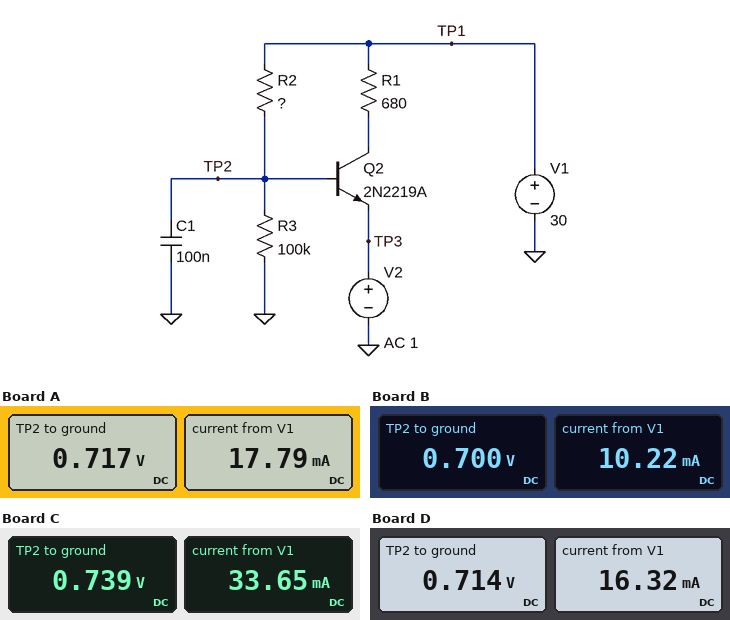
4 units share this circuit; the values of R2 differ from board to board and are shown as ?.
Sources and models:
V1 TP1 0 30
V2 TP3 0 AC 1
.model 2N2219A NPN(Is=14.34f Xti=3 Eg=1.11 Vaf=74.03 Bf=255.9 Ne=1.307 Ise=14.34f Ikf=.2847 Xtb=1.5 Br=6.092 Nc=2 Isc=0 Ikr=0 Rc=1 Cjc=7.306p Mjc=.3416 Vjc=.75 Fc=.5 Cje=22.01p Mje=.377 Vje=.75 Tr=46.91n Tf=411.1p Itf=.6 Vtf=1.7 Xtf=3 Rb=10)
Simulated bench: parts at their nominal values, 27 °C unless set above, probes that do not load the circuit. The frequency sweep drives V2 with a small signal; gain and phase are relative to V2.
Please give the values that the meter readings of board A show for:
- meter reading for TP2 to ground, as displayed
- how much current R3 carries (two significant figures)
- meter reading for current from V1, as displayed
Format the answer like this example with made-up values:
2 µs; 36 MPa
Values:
0.717 V; 7.2 µA; 17.79 mA
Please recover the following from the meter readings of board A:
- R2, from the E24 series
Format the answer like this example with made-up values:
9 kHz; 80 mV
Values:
330 kΩ
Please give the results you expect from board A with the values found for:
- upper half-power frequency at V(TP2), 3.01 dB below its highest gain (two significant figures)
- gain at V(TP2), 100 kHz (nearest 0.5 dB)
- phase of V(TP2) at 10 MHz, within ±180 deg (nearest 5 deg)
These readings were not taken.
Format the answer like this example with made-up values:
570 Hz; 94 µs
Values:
4.5 kHz; -26.5 dB; -40 deg
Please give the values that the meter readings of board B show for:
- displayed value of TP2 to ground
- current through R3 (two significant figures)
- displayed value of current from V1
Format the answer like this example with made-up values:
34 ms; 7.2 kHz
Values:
0.700 V; 7.0 µA; 10.22 mA
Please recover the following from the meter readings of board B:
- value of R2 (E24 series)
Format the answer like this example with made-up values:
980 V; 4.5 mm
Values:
560 kΩ
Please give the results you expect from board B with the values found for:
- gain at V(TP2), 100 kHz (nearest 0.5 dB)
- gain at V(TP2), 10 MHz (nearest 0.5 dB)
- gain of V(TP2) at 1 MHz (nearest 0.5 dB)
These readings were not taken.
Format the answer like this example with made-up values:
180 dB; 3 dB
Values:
-31.5 dB; -44.0 dB; -42.5 dB
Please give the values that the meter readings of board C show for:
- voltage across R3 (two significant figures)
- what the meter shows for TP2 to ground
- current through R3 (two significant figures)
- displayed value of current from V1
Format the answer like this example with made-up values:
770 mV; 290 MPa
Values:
740 mV; 0.739 V; 7.4 µA; 33.65 mA
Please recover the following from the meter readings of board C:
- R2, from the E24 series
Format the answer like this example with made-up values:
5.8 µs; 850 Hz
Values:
160 kΩ
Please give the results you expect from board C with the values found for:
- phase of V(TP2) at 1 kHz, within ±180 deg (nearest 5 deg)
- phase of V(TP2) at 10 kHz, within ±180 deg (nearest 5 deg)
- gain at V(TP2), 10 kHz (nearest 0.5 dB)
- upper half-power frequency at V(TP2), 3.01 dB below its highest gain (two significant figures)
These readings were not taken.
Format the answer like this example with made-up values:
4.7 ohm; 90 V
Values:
-5 deg; -45 deg; -3.5 dB; 9.4 kHz
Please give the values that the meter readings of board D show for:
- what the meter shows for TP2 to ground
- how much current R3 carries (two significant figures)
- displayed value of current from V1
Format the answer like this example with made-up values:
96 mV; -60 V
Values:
0.714 V; 7.1 µA; 16.32 mA
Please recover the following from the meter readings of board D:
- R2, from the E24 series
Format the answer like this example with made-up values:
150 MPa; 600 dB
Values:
360 kΩ
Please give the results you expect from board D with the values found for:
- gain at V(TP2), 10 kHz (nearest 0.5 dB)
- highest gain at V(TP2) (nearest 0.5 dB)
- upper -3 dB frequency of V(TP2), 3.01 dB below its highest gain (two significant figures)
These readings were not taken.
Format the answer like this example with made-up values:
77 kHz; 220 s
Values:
-8.5 dB; 0 dB; 4.1 kHz
